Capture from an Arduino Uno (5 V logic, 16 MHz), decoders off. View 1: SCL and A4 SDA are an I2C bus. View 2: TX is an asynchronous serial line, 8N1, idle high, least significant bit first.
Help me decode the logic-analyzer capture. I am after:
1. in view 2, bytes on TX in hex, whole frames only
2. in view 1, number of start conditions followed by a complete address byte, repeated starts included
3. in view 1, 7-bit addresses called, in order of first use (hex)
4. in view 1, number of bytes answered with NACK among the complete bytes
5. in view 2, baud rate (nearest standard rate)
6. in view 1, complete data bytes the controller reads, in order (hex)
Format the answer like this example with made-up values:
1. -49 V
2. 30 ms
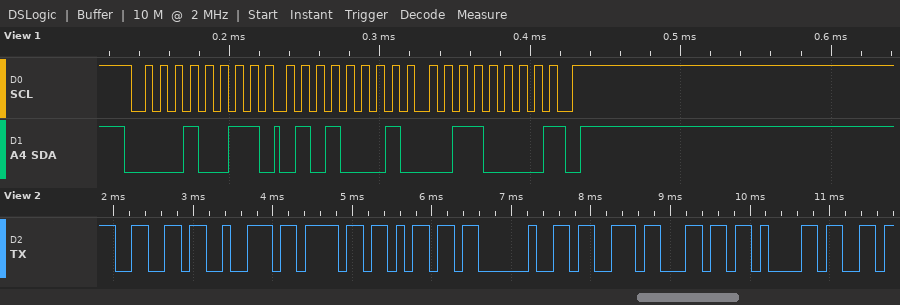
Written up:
1. 0x66 0x72 0x6F 0x6D 0x20 0x73 0x6C 0x61
2. 1
3. 0x09
4. 1
5. 9600 baud
6. 51 30
